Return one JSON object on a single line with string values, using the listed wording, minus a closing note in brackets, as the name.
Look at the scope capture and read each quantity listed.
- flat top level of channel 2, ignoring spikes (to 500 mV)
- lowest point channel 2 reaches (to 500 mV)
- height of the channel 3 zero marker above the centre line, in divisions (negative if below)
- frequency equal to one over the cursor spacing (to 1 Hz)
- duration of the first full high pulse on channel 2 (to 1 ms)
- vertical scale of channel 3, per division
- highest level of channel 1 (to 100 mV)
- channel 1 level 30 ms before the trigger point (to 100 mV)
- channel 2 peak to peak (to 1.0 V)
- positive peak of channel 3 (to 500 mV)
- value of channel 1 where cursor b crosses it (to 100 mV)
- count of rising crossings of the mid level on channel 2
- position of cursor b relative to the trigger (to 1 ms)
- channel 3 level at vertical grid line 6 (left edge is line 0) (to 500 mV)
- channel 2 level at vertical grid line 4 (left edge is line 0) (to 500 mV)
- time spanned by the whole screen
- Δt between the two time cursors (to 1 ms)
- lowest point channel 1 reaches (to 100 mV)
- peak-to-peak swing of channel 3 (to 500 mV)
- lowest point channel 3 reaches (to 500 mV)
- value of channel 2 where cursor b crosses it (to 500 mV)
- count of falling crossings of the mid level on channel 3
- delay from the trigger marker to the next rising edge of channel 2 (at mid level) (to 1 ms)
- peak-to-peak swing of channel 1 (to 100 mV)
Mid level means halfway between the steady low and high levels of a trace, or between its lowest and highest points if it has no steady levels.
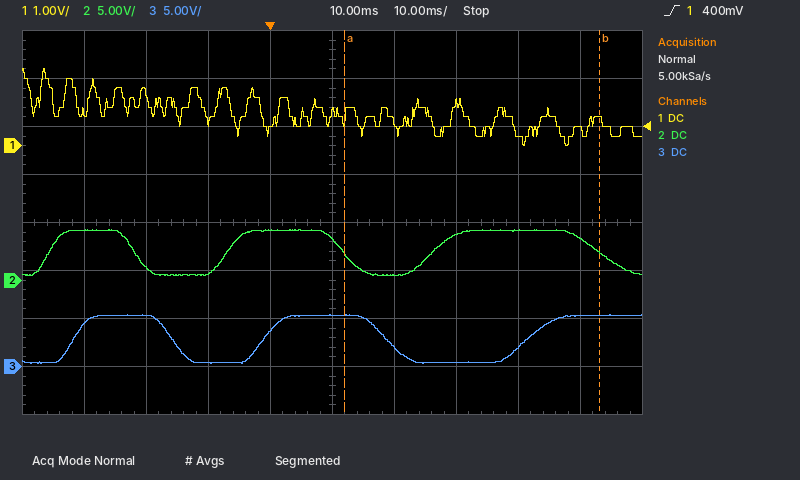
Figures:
{"flat top level of channel 2, ignoring spikes": "5.0 V", "lowest point channel 2 reaches": "500 mV", "height of the channel 3 zero marker above the centre line, in divisions": "-3.0 div", "frequency equal to one over the cursor spacing": "24 Hz", "duration of the first full high pulse on channel 2": "14 ms", "vertical scale of channel 3, per division": "5 V", "highest level of channel 1": "1.6 V", "channel 1 level 30 ms before the trigger point": "700 mV", "channel 2 peak to peak": "5.0 V", "positive peak of channel 3": "5.5 V", "value of channel 1 where cursor b crosses it": "500 mV", "count of rising crossings of the mid level on channel 2": "3", "position of cursor b relative to the trigger": "+53 ms", "channel 3 level at vertical grid line 6 (left edge is line 0)": "2.0 V", "channel 2 level at vertical grid line 4 (left edge is line 0)": "5.0 V", "time spanned by the whole screen": "100 ms", "Δt between the two time cursors": "41 ms", "lowest point channel 1 reaches": "0.0 V", "peak-to-peak swing of channel 3": "5.0 V", "lowest point channel 3 reaches": "500 mV", "value of channel 2 where cursor b crosses it": "3.0 V", "count of falling crossings of the mid level on channel 3": "2", "delay from the trigger marker to the next rising edge of channel 2 (at mid level)": "26 ms", "peak-to-peak swing of channel 1": "1.6 V"}
